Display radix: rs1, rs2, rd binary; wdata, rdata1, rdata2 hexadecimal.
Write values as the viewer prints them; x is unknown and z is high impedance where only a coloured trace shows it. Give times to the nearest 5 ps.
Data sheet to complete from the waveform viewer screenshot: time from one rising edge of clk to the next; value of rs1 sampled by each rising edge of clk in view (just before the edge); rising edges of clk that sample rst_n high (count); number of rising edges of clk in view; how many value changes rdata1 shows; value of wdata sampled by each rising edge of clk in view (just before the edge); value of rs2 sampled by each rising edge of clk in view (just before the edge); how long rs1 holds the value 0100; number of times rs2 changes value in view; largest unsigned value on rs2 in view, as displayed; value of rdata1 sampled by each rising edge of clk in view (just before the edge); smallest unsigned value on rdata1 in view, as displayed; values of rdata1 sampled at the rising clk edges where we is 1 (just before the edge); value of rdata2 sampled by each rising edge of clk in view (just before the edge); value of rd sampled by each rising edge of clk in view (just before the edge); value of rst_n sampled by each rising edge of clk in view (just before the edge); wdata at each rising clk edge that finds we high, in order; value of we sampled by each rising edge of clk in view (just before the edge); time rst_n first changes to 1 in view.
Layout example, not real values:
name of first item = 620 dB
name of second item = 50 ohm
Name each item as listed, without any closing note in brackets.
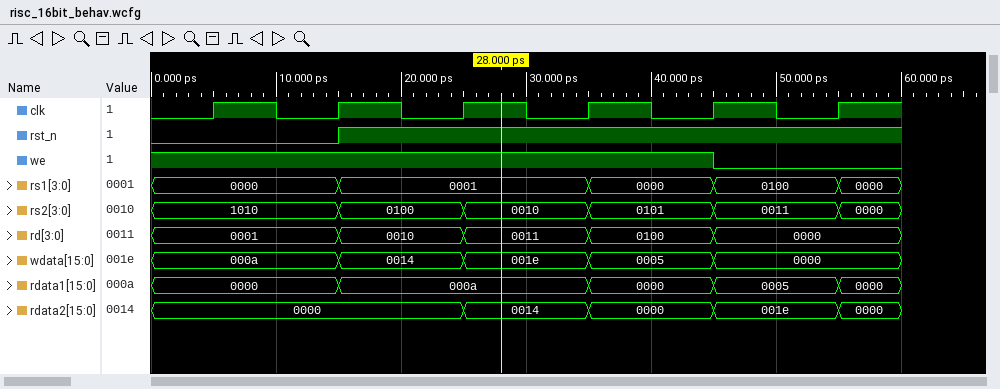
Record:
time from one rising edge of clk to the next = 10 ps
value of rs1 sampled by each rising edge of clk in view = 0000, 0000, 0001, 0001, 0000, 0100
rising edges of clk that sample rst_n high = 4
number of rising edges of clk in view = 6
how many value changes rdata1 shows = 4
value of wdata sampled by each rising edge of clk in view = 000a, 000a, 0014, 001e, 0005, 0000
value of rs2 sampled by each rising edge of clk in view = 1010, 1010, 0100, 0010, 0101, 0011
how long rs1 holds the value 0100 = 10 ps
number of times rs2 changes value in view = 5
largest unsigned value on rs2 in view, as displayed = 1010
value of rdata1 sampled by each rising edge of clk in view = 0000, 0000, 000a, 000a, 0000, 0005
smallest unsigned value on rdata1 in view, as displayed = 0000
values of rdata1 sampled at the rising clk edges where we is 1 = 0000, 0000, 000a, 000a, 0000
value of rdata2 sampled by each rising edge of clk in view = 0000, 0000, 0000, 0014, 0000, 001e
value of rd sampled by each rising edge of clk in view = 0001, 0001, 0010, 0011, 0100, 0000
value of rst_n sampled by each rising edge of clk in view = 0 0 1 1 1 1
wdata at each rising clk edge that finds we high, in order = 000a, 000a, 0014, 001e, 0005
value of we sampled by each rising edge of clk in view = 1 1 1 1 1 0
time rst_n first changes to 1 in view = 15 ps
